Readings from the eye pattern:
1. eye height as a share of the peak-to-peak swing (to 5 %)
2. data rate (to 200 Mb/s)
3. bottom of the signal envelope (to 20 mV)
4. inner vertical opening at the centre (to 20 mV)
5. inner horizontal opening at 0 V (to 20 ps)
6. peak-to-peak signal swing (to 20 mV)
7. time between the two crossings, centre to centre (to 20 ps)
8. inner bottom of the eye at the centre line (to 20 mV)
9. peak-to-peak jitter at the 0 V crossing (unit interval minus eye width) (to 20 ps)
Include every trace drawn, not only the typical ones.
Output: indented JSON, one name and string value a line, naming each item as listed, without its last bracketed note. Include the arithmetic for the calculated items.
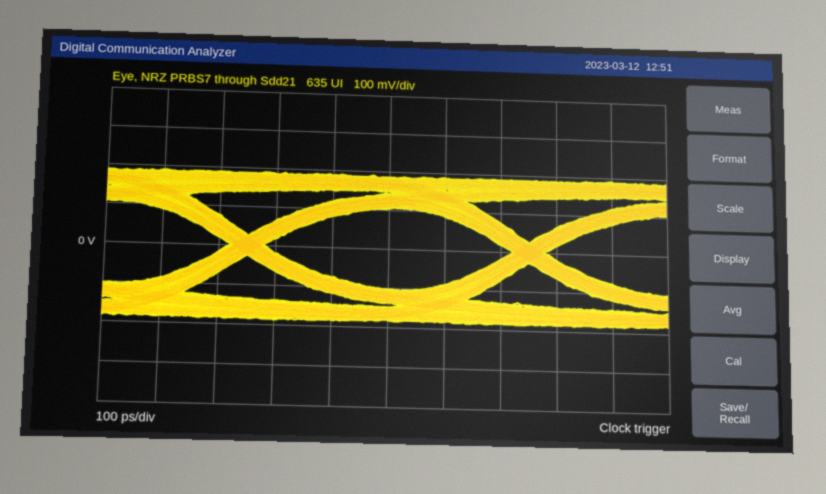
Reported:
{
  "eye height as a share of the peak-to-peak swing": "200 mV / 380 mV ≈ 52.6 %, so 55 % to the nearest 5 %",
  "data rate": "2.0 Gb/s",
  "bottom of the signal envelope": "-180 mV",
  "inner vertical opening at the centre": "200 mV",
  "inner horizontal opening at 0 V": "440 ps",
  "peak-to-peak signal swing": "380 mV",
  "time between the two crossings, centre to centre": "500 ps",
  "inner bottom of the eye at the centre line": "-100 mV",
  "peak-to-peak jitter at the 0 V crossing (unit interval minus eye width)": "60 ps"
}
